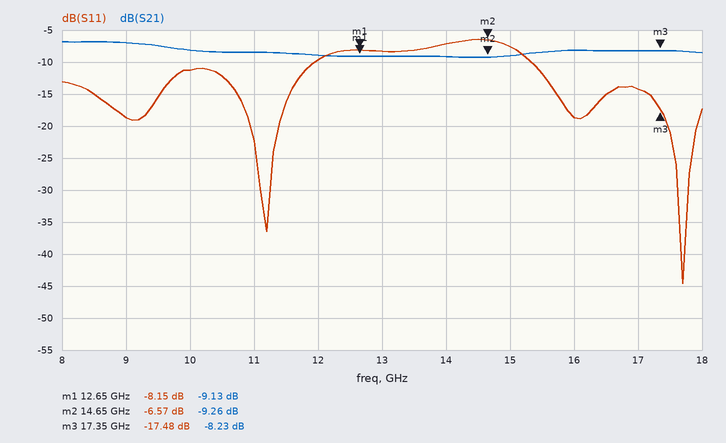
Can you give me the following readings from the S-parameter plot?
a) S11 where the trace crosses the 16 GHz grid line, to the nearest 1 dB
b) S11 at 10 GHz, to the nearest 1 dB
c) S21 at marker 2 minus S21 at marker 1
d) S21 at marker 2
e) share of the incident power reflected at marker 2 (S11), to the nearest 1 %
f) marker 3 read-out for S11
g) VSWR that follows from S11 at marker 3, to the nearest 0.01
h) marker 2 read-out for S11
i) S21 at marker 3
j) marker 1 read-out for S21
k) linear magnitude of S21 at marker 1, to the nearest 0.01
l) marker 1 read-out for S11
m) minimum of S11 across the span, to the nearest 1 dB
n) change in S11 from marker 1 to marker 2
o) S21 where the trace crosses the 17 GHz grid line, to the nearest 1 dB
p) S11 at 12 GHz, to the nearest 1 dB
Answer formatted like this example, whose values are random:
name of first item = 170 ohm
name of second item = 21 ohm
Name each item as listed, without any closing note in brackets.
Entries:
S11 where the trace crosses the 16 GHz grid line, to the nearest 1 dB = -19 dB
S11 at 10 GHz, to the nearest 1 dB = -11 dB
S21 at marker 2 minus S21 at marker 1 = -0.13 dB
S21 at marker 2 = -9.26 dB
share of the incident power reflected at marker 2 (S11), to the nearest 1 % = 22 %
marker 3 read-out for S11 = -17.48 dB
VSWR that follows from S11 at marker 3, to the nearest 0.01 = 1.31
marker 2 read-out for S11 = -6.57 dB
S21 at marker 3 = -8.23 dB
marker 1 read-out for S21 = -9.13 dB
linear magnitude of S21 at marker 1, to the nearest 0.01 = 0.35
marker 1 read-out for S11 = -8.15 dB
minimum of S11 across the span, to the nearest 1 dB = -45 dB
change in S11 from marker 1 to marker 2 = 1.58 dB
S21 where the trace crosses the 17 GHz grid line, to the nearest 1 dB = -8 dB
S11 at 12 GHz, to the nearest 1 dB = -10 dB
